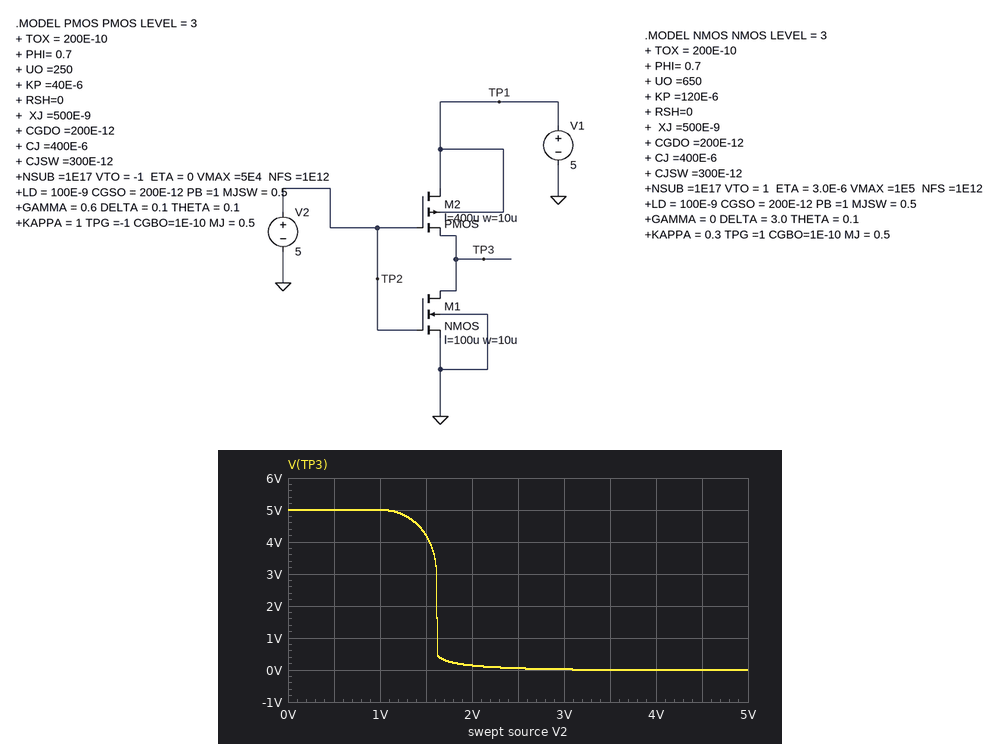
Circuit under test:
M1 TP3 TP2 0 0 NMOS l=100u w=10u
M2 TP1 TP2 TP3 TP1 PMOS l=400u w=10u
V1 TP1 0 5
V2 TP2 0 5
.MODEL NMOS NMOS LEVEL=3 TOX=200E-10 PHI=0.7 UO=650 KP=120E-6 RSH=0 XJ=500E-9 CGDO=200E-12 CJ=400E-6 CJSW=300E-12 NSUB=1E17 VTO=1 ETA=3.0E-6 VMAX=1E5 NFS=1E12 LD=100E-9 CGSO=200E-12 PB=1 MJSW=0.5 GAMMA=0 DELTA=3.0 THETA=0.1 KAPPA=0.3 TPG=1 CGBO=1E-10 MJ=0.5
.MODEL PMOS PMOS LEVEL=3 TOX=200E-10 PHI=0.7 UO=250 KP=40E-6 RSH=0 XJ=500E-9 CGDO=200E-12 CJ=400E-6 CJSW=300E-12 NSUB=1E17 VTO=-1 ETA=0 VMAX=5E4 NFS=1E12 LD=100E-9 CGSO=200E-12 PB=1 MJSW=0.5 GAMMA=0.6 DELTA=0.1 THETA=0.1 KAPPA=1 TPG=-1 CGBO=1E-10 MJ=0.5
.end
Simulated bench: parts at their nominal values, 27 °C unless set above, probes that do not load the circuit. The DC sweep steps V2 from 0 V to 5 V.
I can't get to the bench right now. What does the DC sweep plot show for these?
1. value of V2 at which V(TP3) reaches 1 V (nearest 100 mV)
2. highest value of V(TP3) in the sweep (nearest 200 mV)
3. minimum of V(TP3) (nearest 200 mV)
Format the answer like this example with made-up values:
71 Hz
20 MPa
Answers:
1.6 V
5.0 V
0 V
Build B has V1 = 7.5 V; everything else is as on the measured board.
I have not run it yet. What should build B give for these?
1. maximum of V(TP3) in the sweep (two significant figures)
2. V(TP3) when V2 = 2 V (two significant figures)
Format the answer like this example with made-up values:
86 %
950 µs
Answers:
7.5 V
5.1 V
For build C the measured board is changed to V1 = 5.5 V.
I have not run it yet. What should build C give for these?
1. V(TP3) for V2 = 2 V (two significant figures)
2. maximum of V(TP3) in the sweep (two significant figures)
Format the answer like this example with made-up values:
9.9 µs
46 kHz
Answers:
220 mV
5.5 V
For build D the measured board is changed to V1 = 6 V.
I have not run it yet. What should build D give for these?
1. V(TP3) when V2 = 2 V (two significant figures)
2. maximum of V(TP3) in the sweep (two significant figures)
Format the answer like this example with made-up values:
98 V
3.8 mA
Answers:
330 mV
6.0 V
